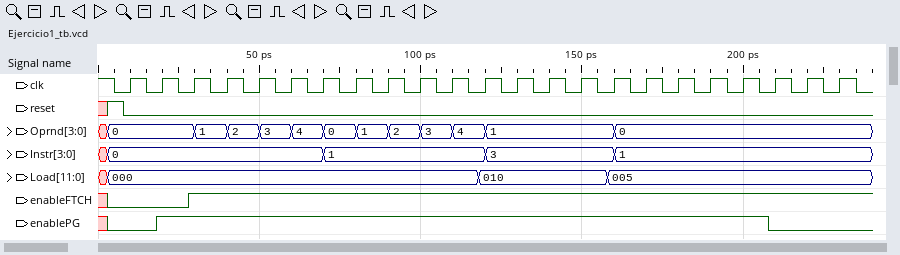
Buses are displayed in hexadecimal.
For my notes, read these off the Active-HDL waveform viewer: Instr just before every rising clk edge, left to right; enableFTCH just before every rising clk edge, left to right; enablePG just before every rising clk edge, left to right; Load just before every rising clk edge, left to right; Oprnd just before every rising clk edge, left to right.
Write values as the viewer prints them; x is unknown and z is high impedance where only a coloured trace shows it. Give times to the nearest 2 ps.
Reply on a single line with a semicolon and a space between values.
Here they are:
0, 0, 0, 0, 0, 0, 0, 1, 1, 1, 1, 1, 3, 3, 3, 3, 1, 1, 1, 1, 1, 1, 1; 0 0 1 1 1 1 1 1 1 1 1 1 1 1 1 1 1 1 1 1 1 1 1; 0 1 1 1 1 1 1 1 1 1 1 1 1 1 1 1 1 1 1 1 0 0 0; 000, 000, 000, 000, 000, 000, 000, 000, 000, 000, 000, 010, 010, 010, 010, 005, 005, 005, 005, 005, 005, 005, 005; 0, 0, 0, 1, 2, 3, 4, 0, 1, 2, 3, 4, 1, 1, 1, 1, 0, 0, 0, 0, 0, 0, 0
